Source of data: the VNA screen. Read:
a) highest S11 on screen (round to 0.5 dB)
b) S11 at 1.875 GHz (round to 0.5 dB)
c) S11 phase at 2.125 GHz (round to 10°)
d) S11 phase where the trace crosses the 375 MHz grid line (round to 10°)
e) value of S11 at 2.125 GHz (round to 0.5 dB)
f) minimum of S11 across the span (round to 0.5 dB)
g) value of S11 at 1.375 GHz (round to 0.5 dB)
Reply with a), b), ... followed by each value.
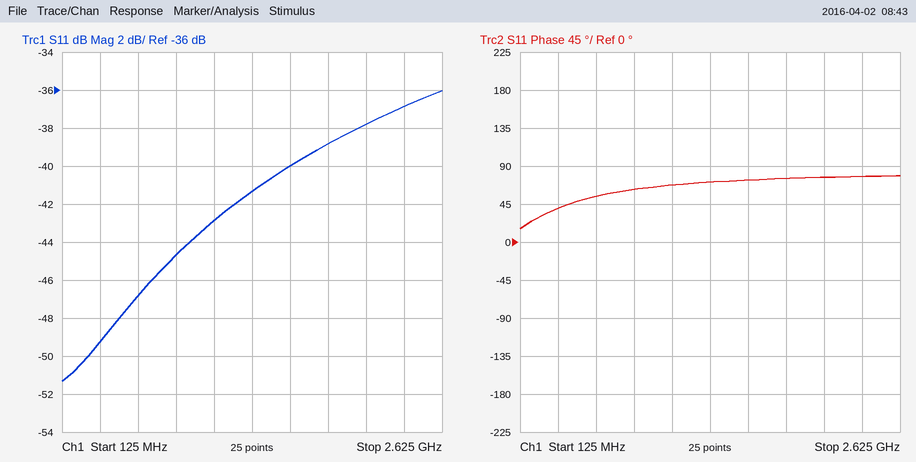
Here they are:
a) -36.0 dB
b) -39.0 dB
c) 80°
d) 40°
e) -38.0 dB
f) -51.5 dB
g) -41.5 dB
